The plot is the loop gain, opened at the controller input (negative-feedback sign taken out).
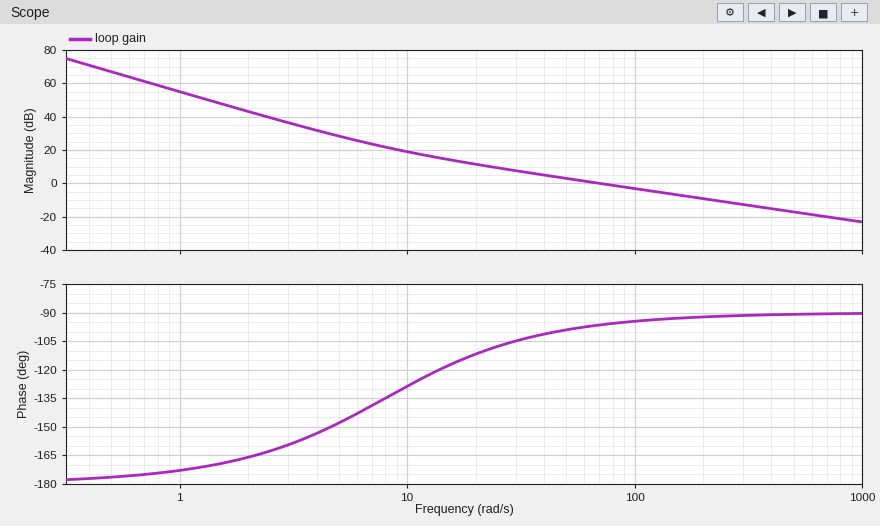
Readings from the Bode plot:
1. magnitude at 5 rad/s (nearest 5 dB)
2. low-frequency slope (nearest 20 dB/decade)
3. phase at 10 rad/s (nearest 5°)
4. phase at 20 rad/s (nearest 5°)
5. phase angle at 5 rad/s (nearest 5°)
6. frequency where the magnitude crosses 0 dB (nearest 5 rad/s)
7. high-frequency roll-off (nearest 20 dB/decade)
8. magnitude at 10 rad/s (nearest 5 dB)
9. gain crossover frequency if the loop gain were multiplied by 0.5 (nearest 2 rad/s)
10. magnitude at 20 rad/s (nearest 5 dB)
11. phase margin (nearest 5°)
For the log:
30 dB
-40 dB/decade
-130°
-110°
-150°
70 rad/s
-20 dB/decade
20 dB
36 rad/s
10 dB
85°
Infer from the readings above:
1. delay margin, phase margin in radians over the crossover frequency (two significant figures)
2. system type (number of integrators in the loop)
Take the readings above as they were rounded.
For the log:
0.021 s
2
